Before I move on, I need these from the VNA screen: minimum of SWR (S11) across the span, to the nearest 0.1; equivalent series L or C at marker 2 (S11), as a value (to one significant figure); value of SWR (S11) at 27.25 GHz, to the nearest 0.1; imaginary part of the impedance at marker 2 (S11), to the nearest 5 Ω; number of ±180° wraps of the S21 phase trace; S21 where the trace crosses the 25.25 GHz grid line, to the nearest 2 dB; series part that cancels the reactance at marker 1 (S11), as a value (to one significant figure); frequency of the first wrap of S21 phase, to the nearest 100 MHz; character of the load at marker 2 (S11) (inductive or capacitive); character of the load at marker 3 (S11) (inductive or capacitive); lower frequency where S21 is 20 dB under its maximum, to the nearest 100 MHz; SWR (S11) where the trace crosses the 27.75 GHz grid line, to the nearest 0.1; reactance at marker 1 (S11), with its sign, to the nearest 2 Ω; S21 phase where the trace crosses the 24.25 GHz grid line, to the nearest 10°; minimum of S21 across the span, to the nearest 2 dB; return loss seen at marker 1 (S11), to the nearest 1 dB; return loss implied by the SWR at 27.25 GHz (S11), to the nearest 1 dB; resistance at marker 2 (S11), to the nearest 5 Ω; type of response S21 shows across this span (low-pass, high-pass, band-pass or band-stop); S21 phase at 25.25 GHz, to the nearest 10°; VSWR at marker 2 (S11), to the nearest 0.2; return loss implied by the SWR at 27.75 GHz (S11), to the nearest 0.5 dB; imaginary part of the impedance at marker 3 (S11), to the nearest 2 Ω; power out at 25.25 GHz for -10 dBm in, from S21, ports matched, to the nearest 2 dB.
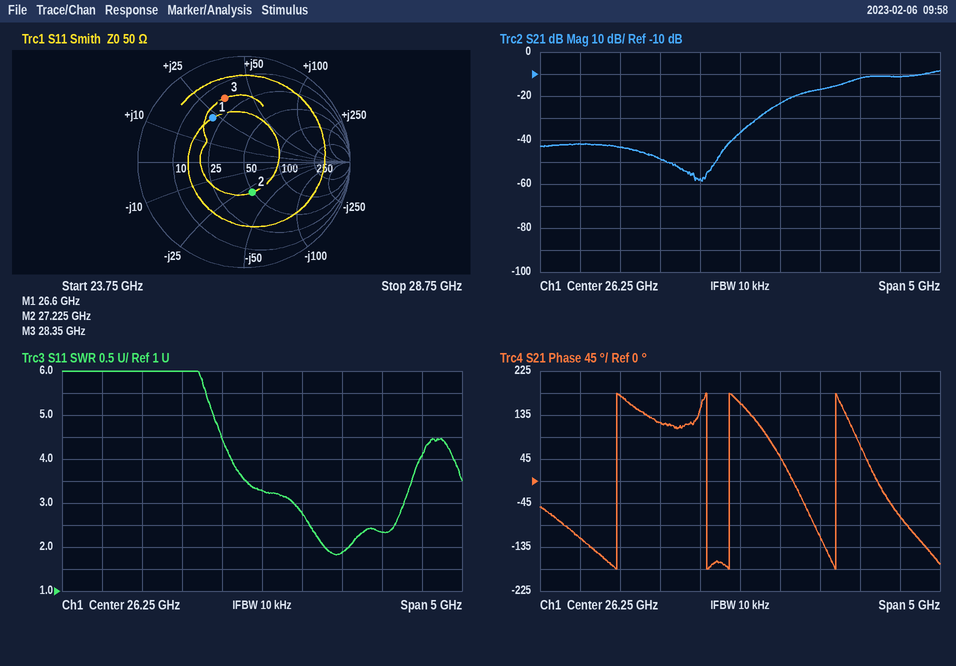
1.8
200 fF
1.9
-30 Ω
4
-48 dB
300 fF
24.7 GHz
capacitive
inductive
26.5 GHz
2.3
+22 Ω
-120°
-58 dB
6 dB
10 dB
50 Ω
high-pass
120°
1.8
8.0 dB
+34 Ω
-58 dBm
